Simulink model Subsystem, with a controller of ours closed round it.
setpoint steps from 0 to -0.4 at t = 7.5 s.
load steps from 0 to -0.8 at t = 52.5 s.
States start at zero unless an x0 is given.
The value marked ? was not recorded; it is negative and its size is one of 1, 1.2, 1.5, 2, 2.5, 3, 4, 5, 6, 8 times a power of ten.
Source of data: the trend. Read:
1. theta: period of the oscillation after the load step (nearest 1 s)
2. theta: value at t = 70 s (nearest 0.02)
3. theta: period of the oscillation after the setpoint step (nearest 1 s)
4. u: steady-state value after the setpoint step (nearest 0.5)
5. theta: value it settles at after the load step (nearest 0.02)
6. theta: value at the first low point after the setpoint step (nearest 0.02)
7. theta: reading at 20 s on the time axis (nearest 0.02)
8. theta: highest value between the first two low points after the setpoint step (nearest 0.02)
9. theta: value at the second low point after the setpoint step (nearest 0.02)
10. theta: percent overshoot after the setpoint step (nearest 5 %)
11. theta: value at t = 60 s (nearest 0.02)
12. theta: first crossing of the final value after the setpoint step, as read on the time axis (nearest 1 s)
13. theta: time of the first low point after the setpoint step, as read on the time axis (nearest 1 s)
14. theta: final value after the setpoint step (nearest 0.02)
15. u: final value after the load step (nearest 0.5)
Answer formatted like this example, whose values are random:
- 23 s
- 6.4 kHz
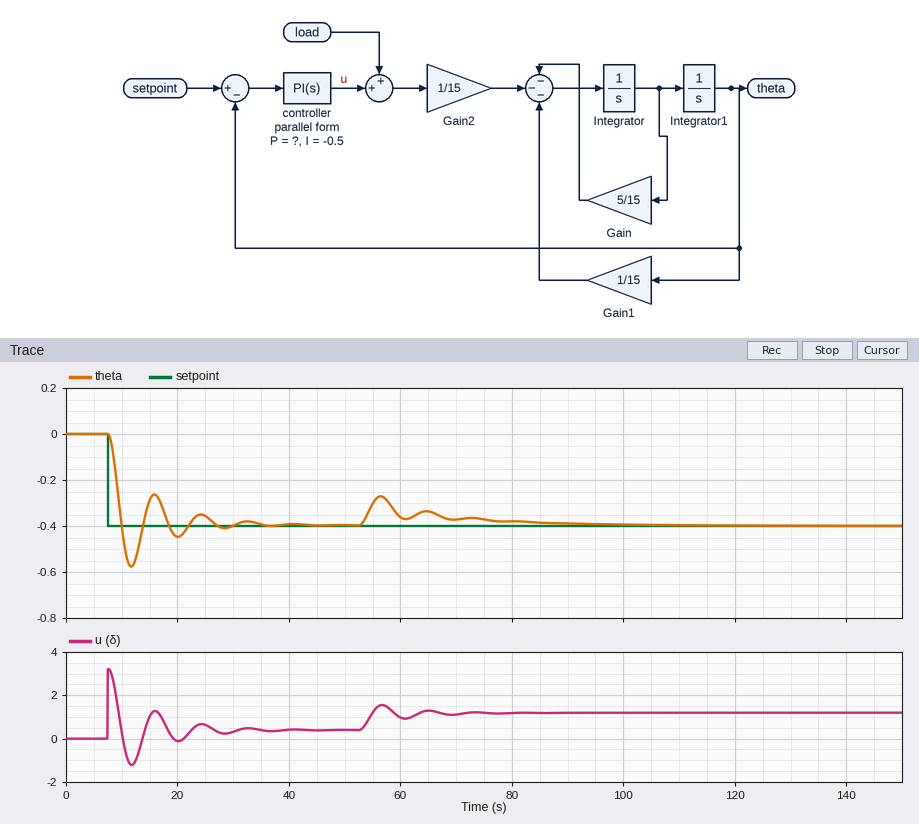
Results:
- 8 s
- -0.38
- 8 s
- 0.5
- -0.40
- -0.58
- -0.44
- -0.26
- -0.44
- 45 %
- -0.36
- 10 s
- 12 s
- -0.40
- 1.0
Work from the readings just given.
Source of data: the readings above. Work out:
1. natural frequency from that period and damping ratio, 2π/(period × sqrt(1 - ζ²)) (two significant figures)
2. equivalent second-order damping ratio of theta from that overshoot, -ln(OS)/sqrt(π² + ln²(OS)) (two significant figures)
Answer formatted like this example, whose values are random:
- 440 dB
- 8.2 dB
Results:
- 0.81 rad/s
- 0.25
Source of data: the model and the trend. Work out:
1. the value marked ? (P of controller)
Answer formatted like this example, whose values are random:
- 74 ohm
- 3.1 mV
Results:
- -8
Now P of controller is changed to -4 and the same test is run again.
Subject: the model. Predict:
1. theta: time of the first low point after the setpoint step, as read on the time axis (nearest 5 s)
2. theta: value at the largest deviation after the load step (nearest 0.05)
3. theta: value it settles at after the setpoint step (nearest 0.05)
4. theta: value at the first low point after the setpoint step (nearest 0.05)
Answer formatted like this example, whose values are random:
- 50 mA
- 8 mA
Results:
- 15 s
- -0.20
- -0.40
- -0.55
